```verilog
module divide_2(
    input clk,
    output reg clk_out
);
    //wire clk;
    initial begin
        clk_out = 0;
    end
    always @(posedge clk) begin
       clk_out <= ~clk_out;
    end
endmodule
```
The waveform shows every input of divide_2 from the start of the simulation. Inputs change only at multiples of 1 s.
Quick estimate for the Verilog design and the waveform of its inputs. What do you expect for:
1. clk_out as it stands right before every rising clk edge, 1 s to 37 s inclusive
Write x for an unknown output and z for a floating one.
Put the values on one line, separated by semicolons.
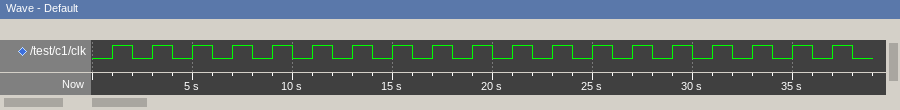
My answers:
0 1 0 1 0 1 0 1 0 1 0 1 0 1 0 1 0 1 0
